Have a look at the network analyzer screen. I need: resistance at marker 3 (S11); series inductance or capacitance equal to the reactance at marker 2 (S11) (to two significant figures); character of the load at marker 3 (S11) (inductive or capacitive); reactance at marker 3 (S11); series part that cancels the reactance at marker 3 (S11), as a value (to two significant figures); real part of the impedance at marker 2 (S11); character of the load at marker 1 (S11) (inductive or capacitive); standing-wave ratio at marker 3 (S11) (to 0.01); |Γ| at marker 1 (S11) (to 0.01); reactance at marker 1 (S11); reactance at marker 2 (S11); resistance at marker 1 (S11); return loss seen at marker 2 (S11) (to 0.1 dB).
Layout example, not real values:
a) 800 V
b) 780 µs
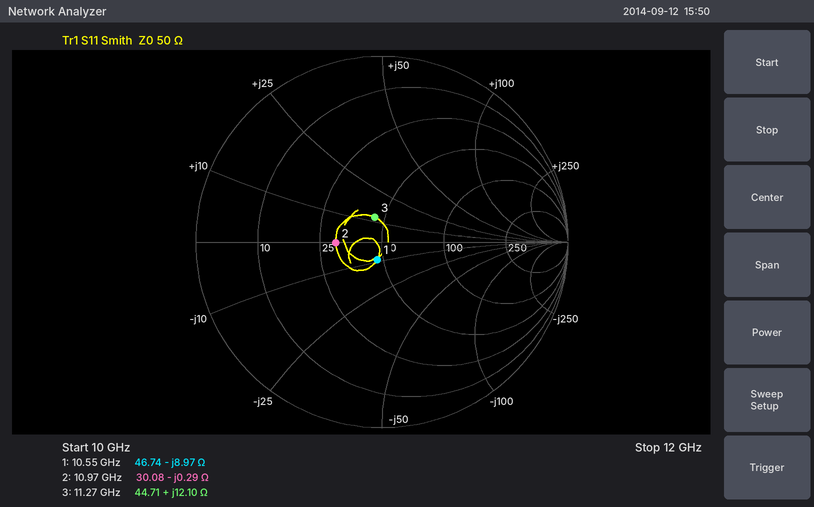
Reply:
a) 44.71 Ω
b) 50 pF
c) inductive
d) +12.10 Ω
e) 1.2 pF
f) 30.08 Ω
g) capacitive
h) 1.32
i) 0.10
j) -8.97 Ω
k) -0.29 Ω
l) 46.74 Ω
m) 12.1 dB
